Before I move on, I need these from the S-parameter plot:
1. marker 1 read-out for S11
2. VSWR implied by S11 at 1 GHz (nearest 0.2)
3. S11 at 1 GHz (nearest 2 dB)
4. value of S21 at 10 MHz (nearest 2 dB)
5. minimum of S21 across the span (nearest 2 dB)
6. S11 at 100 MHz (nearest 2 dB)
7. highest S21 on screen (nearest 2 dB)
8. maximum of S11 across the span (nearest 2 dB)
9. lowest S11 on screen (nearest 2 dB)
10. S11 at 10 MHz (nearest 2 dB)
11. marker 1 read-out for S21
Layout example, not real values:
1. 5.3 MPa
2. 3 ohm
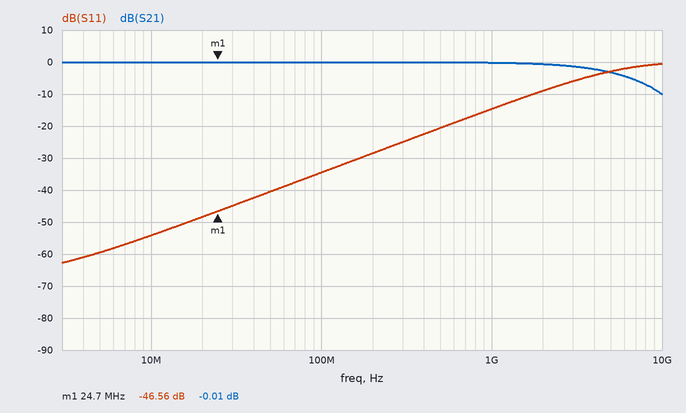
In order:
1. -46.56 dB
2. 1.4
3. -14 dB
4. 0 dB
5. -10 dB
6. -34 dB
7. 0 dB
8. 0 dB
9. -62 dB
10. -54 dB
11. -0.01 dB
